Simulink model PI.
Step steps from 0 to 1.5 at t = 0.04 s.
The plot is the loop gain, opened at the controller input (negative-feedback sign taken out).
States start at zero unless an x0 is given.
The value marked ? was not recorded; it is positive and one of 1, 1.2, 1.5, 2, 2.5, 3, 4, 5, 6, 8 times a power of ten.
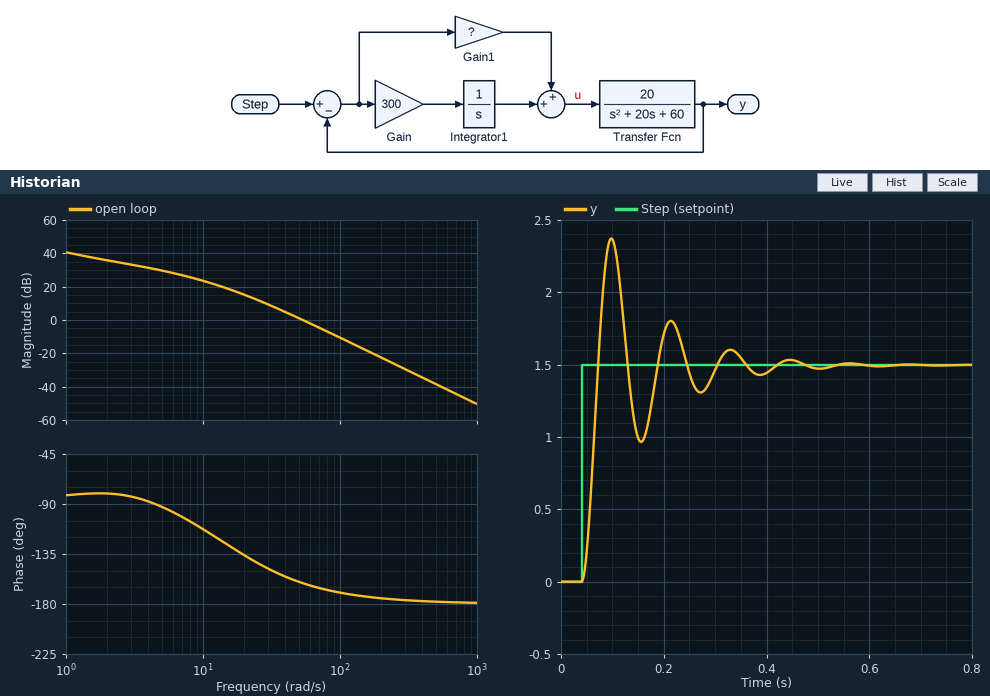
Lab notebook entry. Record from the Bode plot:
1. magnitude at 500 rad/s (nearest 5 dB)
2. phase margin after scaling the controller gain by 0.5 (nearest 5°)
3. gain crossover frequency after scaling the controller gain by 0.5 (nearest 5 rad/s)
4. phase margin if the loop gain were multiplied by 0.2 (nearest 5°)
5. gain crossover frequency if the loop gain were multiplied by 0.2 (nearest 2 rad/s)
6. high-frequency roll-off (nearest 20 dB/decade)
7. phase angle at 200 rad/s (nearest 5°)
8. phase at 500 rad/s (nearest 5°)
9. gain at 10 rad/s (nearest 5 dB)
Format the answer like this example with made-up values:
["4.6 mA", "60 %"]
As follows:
["-40 dB", "25°", "35 rad/s", "40°", "22 rad/s", "-40 dB/decade", "-175°", "-180°", "25 dB"]
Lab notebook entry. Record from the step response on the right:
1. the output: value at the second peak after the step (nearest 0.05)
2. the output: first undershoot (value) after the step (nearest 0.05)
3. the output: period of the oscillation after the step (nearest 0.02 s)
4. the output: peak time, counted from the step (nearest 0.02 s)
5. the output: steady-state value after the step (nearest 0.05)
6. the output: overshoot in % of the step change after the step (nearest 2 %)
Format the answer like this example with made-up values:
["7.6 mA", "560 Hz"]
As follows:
["1.80", "0.95", "0.12 s", "0.06 s", "1.50", "58 %"]
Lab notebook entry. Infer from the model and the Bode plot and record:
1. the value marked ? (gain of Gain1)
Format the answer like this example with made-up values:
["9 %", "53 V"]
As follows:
["150"]
